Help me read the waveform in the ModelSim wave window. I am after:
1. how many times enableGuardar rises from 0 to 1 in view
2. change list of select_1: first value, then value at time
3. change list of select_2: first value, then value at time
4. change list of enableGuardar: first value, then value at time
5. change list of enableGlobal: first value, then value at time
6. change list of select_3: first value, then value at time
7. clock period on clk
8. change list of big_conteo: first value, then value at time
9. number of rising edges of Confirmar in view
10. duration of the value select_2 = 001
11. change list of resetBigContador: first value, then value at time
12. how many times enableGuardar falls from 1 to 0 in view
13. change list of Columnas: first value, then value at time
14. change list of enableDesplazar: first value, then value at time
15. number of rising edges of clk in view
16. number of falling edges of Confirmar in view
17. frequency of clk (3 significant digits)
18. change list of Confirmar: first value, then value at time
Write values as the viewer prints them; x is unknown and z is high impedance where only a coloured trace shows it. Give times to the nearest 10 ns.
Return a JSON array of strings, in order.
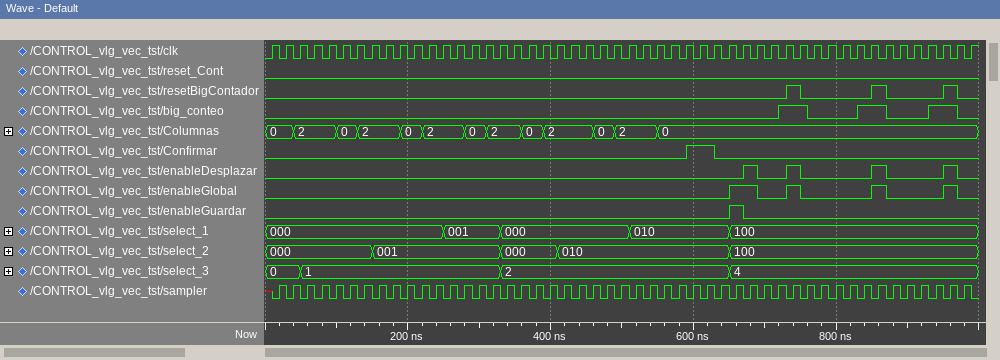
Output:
["1", "000, 001 at 250 ns, 000 at 330 ns, 010 at 510 ns, 100 at 650 ns", "000, 001 at 150 ns, 000 at 330 ns, 010 at 410 ns, 100 at 650 ns", "0, 1 at 650 ns, 0 at 670 ns", "0, 1 at 650 ns, 0 at 690 ns, 1 at 730 ns, 0 at 750 ns, 1 at 850 ns, 0 at 870 ns, 1 at 950 ns, 0 at 970 ns", "0, 1 at 50 ns, 2 at 330 ns, 4 at 650 ns", "20 ns", "0, 1 at 720 ns, 0 at 760 ns, 1 at 830 ns, 0 at 870 ns, 1 at 930 ns, 0 at 970 ns", "1", "180 ns", "0, 1 at 730 ns, 0 at 750 ns, 1 at 850 ns, 0 at 870 ns, 1 at 950 ns, 0 at 970 ns", "1", "0, 2 at 40 ns, 0 at 100 ns, 2 at 130 ns, 0 at 190 ns, 2 at 220 ns, 0 at 280 ns, 2 at 310 ns, 0 at 360 ns, 2 at 390 ns, 0 at 460 ns, 2 at 490 ns, 0 at 550 ns", "0, 1 at 670 ns, 0 at 690 ns, 1 at 730 ns, 0 at 750 ns, 1 at 850 ns, 0 at 870 ns, 1 at 950 ns, 0 at 970 ns", "50", "1", "50.0 MHz", "0, 1 at 590 ns, 0 at 630 ns"]
